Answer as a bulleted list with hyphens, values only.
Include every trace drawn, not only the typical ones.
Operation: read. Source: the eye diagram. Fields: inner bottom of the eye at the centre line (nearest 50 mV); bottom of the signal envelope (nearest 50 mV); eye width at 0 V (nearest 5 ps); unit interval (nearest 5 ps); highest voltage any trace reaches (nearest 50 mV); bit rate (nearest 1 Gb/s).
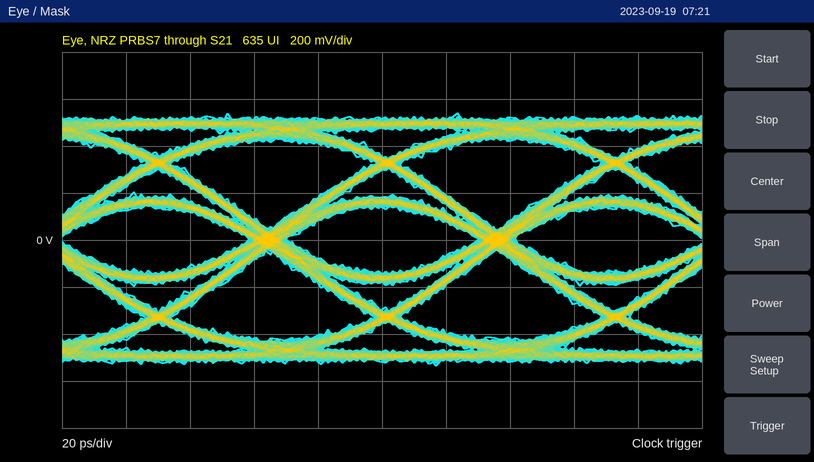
- -150 mV
- -550 mV
- 60 ps
- 70 ps
- 550 mV
- 14 Gb/s
